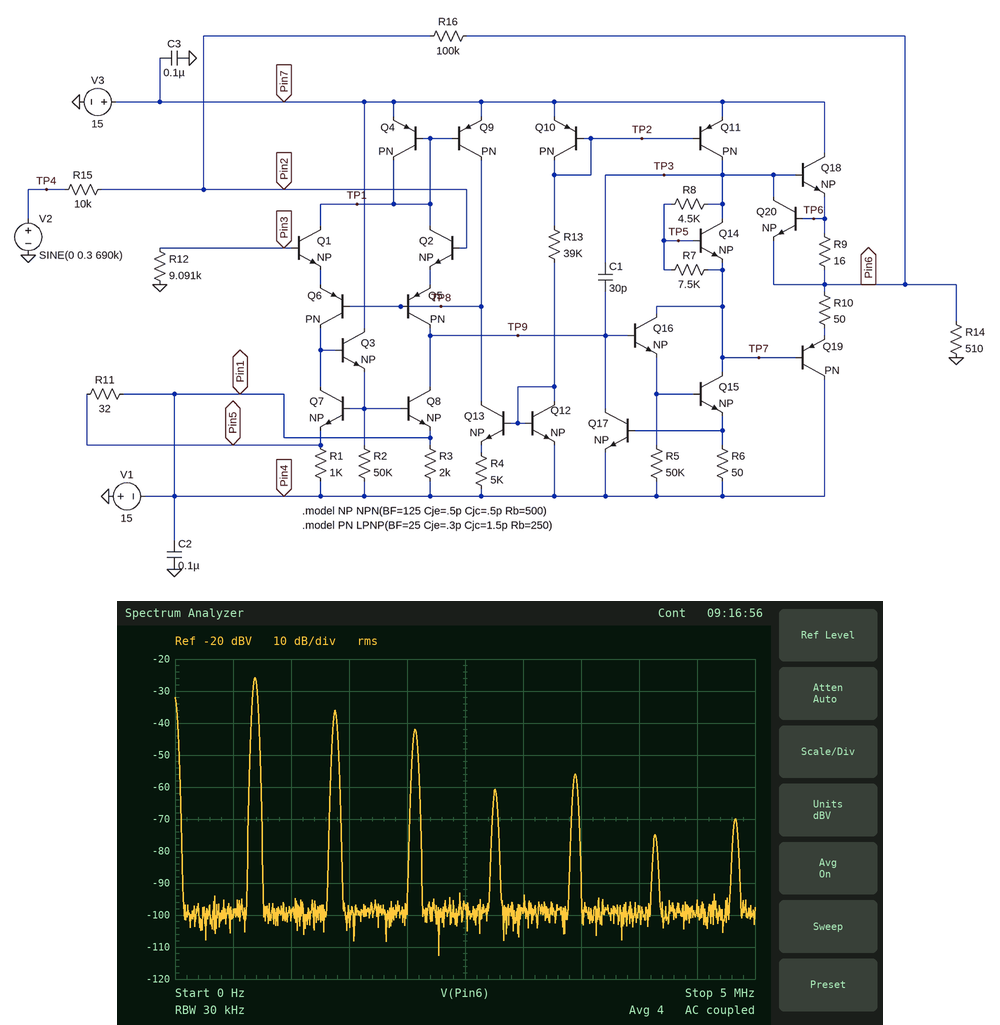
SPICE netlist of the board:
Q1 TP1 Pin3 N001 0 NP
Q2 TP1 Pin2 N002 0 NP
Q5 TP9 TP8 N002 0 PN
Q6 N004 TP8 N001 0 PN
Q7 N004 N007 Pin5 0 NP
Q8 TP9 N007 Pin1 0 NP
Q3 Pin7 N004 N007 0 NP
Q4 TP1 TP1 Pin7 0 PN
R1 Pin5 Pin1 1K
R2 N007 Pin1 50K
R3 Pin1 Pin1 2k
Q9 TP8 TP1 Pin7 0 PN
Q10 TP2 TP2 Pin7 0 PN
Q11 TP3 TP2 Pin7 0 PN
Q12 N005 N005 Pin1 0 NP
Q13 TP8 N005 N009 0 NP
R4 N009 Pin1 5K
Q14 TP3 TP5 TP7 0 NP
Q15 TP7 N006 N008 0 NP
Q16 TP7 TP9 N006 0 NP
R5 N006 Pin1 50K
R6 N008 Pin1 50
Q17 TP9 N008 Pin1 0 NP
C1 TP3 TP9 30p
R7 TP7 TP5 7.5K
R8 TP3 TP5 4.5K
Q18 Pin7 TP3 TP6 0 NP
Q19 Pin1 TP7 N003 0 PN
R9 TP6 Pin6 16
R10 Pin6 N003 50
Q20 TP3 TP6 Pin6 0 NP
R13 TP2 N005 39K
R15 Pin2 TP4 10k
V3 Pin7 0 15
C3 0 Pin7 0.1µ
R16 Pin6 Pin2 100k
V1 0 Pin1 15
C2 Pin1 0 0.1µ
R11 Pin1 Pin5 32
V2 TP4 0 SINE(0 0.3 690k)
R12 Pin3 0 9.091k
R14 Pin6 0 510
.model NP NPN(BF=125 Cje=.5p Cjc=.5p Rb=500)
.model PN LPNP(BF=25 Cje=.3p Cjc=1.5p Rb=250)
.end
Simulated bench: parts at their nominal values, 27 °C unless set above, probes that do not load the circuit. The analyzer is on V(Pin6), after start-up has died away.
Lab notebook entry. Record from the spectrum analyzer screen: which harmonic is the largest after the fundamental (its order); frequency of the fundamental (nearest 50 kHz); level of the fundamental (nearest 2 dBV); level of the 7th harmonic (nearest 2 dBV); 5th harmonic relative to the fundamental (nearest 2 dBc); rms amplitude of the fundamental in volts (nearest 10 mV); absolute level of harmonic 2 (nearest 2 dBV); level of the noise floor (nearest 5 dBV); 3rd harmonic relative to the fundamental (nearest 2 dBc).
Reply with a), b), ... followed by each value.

a) 2
b) 700 kHz
c) -26 dBV
d) -70 dBV
e) -30 dBc
f) 50 mV
g) -36 dBV
h) -100 dBV
i) -16 dBc
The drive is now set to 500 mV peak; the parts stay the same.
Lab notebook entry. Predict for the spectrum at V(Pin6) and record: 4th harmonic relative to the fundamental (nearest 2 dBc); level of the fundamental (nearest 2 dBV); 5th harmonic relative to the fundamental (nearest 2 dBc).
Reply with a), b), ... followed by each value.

a) -42 dBc
b) -26 dBV
c) -26 dBc
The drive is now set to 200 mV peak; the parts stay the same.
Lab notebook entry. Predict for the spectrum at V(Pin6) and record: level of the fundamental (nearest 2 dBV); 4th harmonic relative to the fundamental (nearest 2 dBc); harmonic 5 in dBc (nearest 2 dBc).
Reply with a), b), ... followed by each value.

a) -28 dBV
b) -32 dBc
c) -38 dBc
